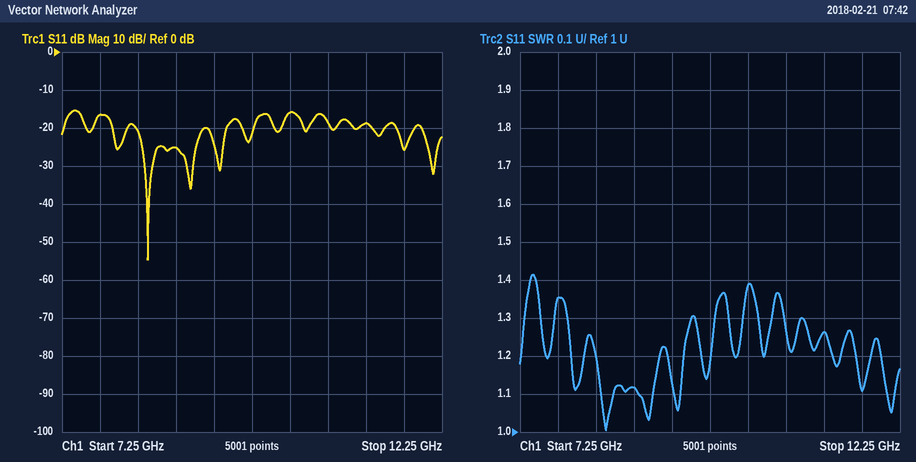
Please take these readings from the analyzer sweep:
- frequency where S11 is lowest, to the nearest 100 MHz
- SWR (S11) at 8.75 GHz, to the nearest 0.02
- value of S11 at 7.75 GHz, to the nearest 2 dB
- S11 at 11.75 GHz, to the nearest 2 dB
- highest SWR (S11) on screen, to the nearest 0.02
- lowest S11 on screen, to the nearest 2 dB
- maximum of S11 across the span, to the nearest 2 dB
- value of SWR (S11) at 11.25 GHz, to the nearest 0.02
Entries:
8.4 GHz
1.12
-16 dB
-26 dB
1.42
-54 dB
-16 dB
1.26
